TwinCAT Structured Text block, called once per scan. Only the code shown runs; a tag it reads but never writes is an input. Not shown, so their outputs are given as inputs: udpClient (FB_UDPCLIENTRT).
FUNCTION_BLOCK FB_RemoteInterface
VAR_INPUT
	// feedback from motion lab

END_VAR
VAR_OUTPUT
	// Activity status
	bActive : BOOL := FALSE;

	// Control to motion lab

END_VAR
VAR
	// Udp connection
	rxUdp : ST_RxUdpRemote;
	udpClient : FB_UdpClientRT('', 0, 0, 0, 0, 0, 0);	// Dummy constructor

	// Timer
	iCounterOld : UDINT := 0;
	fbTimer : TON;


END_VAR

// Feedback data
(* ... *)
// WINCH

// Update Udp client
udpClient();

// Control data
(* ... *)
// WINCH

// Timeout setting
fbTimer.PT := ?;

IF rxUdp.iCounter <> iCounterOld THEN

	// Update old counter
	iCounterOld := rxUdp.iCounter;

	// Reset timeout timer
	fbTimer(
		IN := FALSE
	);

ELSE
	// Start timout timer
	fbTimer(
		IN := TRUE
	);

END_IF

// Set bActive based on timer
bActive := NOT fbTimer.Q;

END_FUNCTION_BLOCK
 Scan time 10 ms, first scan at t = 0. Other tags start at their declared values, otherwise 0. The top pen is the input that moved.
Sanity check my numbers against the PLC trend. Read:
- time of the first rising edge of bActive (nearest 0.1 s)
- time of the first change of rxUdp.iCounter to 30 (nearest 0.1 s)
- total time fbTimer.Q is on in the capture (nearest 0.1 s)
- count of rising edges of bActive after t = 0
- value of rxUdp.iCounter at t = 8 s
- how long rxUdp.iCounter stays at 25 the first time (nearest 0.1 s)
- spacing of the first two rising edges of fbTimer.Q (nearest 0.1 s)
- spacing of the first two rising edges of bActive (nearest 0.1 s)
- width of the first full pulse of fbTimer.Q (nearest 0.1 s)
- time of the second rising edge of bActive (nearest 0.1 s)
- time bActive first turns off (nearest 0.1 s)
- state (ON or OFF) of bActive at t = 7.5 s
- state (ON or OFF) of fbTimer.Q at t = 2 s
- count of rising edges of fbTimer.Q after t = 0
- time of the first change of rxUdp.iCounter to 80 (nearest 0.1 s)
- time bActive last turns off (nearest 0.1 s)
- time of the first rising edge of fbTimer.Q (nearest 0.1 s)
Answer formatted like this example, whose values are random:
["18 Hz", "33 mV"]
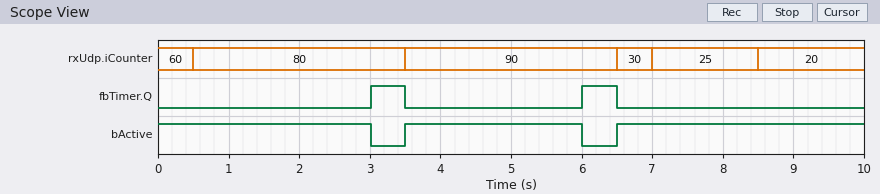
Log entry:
["3.5 s", "6.5 s", "1.0 s", "2", "25", "1.5 s", "3.0 s", "3.0 s", "0.5 s", "6.5 s", "3.0 s", "ON", "OFF", "2", "0.5 s", "6.0 s", "3.0 s"]
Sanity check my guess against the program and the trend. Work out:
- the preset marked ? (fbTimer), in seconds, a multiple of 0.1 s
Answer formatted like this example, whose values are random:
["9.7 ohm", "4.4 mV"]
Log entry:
["2.5 s"]
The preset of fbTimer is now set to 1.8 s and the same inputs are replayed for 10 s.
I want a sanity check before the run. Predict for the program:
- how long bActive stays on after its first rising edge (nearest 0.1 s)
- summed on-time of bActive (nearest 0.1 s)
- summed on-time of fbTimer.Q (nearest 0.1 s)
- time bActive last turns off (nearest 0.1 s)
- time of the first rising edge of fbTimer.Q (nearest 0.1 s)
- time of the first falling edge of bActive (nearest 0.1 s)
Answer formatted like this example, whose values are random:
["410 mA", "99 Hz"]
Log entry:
["1.8 s", "7.6 s", "2.4 s", "5.3 s", "2.3 s", "2.3 s"]
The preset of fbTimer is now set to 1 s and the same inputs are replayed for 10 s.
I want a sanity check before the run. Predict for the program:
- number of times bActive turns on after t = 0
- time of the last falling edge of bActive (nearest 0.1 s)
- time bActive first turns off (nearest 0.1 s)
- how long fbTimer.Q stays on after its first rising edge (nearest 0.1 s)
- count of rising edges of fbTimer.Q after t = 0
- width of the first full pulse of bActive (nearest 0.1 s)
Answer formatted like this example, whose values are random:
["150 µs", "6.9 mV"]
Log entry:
["3", "9.5 s", "1.5 s", "2.0 s", "4", "1.0 s"]
